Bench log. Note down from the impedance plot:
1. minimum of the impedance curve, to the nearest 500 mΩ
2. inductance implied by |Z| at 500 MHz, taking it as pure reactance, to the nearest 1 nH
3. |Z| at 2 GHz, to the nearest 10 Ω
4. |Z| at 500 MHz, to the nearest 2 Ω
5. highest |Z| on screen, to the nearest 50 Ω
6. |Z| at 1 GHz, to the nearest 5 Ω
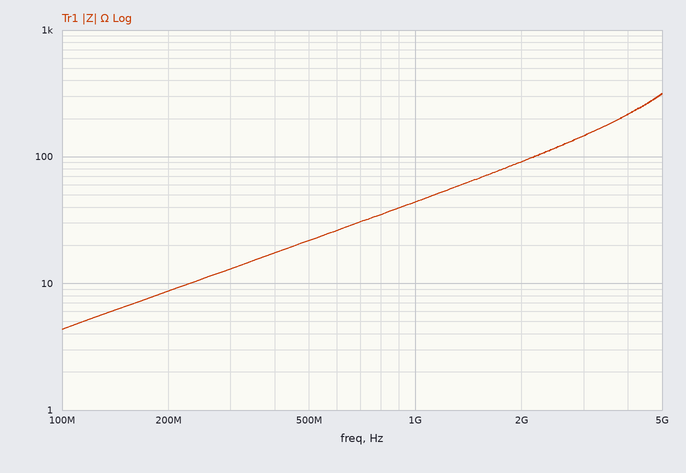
4.5 Ω
7 nH
90 Ω
22 Ω
300 Ω
45 Ω
